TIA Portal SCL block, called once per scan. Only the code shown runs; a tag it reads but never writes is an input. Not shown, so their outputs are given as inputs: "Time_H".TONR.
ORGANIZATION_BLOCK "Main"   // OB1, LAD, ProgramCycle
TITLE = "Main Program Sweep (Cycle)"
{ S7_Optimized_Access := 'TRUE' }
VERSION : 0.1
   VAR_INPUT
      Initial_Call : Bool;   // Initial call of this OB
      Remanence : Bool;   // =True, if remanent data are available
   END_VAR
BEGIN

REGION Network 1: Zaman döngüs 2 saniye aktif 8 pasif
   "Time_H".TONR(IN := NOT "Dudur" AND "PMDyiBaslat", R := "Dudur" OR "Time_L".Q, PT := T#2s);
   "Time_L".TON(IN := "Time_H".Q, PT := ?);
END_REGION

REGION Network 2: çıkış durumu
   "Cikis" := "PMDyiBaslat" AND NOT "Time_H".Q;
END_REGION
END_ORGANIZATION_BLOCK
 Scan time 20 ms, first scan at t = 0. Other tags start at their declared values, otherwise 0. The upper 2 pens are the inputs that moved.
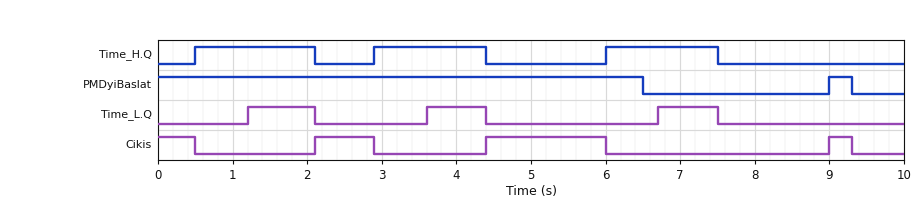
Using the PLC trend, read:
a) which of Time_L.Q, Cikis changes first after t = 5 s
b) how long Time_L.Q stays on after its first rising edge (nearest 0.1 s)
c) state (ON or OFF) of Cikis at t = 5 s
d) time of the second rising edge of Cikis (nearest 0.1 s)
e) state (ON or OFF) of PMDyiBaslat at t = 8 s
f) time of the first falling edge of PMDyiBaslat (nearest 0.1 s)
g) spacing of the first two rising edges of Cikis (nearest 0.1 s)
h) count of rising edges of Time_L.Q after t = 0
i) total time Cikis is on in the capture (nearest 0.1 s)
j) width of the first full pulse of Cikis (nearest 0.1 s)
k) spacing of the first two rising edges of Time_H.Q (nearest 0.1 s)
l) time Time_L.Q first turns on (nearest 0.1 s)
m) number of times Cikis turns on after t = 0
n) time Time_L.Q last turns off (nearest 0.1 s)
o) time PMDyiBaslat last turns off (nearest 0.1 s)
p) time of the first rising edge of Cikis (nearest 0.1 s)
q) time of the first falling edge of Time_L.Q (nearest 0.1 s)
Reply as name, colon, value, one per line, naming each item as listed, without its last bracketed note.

which of Time_L.Q, Cikis changes first after t = 5 s: Cikis
how long Time_L.Q stays on after its first rising edge: 0.9 s
state (ON or OFF) of Cikis at t = 5 s: ON
time of the second rising edge of Cikis: 4.4 s
state (ON or OFF) of PMDyiBaslat at t = 8 s: OFF
time of the first falling edge of PMDyiBaslat: 6.5 s
spacing of the first two rising edges of Cikis: 2.3 s
count of rising edges of Time_L.Q after t = 0: 3
total time Cikis is on in the capture: 3.2 s
width of the first full pulse of Cikis: 0.8 s
spacing of the first two rising edges of Time_H.Q: 2.4 s
time Time_L.Q first turns on: 1.2 s
number of times Cikis turns on after t = 0: 3
time Time_L.Q last turns off: 7.5 s
time PMDyiBaslat last turns off: 9.3 s
time of the first rising edge of Cikis: 2.1 s
time of the first falling edge of Time_L.Q: 2.1 s
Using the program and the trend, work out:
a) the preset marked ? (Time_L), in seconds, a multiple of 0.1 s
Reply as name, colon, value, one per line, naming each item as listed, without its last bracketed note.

the preset marked ? (Time_L), in seconds, a multiple of 0.1 s: 0.7 s
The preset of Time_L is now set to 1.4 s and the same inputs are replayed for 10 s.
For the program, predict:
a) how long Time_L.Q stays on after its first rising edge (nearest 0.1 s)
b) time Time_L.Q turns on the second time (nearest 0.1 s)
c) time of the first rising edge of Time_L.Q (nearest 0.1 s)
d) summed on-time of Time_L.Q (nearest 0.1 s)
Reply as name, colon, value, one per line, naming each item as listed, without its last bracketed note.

how long Time_L.Q stays on after its first rising edge: 0.2 s
time Time_L.Q turns on the second time: 4.3 s
time of the first rising edge of Time_L.Q: 1.9 s
summed on-time of Time_L.Q: 0.4 s
